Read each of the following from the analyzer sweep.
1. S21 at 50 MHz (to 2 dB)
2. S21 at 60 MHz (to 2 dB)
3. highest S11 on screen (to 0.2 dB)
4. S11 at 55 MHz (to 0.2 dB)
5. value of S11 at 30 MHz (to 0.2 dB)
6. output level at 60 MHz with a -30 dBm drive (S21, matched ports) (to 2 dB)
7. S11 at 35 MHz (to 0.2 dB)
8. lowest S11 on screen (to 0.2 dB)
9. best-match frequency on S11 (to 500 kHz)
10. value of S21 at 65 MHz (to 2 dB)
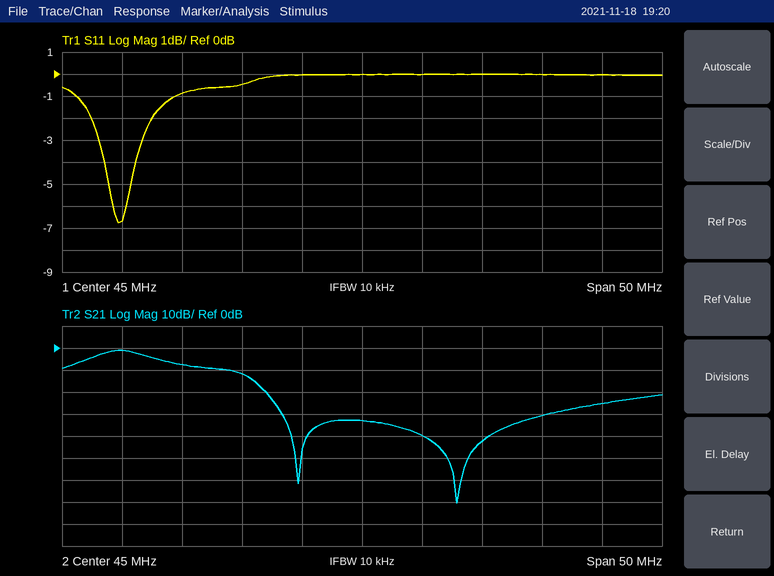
-40 dB
-30 dB
0.0 dB
0.0 dB
-0.8 dB
-60 dBm
-0.4 dB
-6.8 dB
24.5 MHz
-26 dB
